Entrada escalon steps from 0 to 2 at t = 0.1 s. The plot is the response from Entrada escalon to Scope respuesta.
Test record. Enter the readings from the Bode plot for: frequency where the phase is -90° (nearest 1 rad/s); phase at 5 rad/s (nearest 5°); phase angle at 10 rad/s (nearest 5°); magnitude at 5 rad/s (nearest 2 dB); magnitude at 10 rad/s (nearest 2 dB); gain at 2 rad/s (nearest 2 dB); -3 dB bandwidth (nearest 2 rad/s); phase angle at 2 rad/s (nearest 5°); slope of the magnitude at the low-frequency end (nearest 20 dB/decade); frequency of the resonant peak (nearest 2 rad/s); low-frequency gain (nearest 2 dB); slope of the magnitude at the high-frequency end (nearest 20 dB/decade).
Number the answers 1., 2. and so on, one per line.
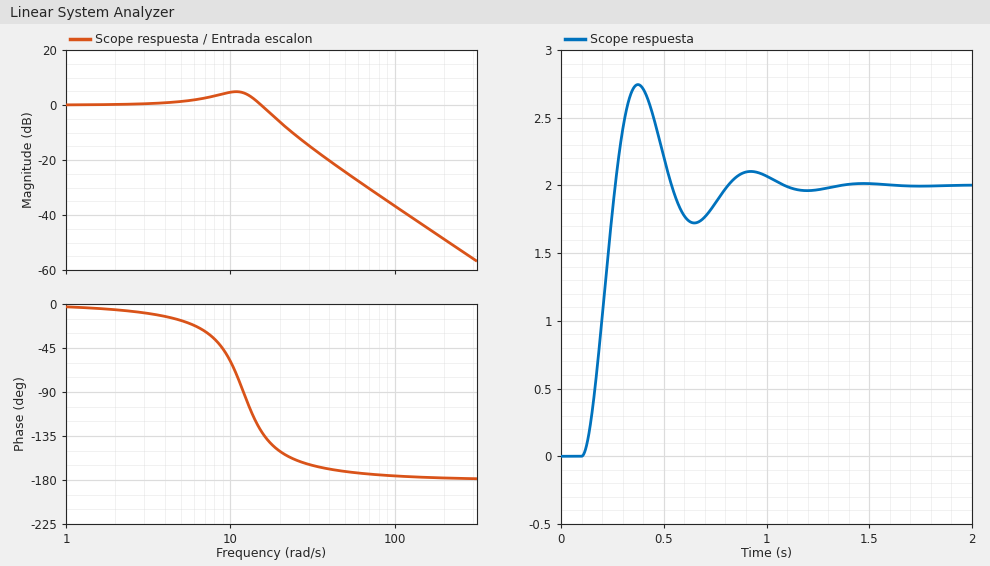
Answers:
1. 12 rad/s
2. -15°
3. -60°
4. 2 dB
5. 4 dB
6. 0 dB
7. 18 rad/s
8. -5°
9. 0 dB/decade
10. 10 rad/s
11. 0 dB
12. -40 dB/decade
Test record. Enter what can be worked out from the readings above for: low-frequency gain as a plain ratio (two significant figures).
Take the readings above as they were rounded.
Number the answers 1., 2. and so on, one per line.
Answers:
1. 1.0
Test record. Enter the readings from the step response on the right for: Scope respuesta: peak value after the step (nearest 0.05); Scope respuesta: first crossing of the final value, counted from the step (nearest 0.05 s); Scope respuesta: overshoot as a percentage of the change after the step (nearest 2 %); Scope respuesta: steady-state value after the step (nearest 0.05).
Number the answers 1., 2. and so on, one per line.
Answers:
1. 2.75
2. 0.15 s
3. 38 %
4. 2.00
